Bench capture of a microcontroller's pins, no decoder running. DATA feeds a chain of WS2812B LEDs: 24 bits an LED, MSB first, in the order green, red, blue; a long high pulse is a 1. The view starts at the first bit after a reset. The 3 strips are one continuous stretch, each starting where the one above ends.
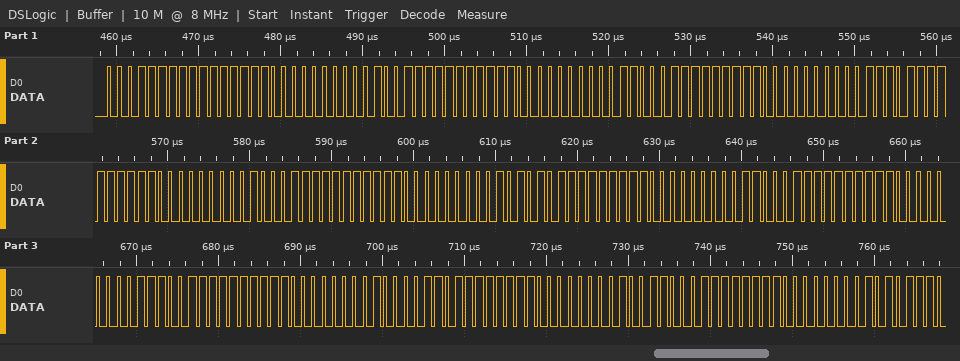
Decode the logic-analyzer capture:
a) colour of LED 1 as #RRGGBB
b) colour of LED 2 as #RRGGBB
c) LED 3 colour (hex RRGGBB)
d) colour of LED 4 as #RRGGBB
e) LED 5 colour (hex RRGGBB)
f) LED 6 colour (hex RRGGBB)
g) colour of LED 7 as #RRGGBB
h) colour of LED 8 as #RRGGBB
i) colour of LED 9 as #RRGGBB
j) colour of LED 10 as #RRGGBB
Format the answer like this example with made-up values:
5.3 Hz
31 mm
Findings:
#FF1F00
#FF2700
#FF3100
#FF3B00
#FF4700
#FF5500
#FF6300
#FF7300
#FF8600
#FF9800
